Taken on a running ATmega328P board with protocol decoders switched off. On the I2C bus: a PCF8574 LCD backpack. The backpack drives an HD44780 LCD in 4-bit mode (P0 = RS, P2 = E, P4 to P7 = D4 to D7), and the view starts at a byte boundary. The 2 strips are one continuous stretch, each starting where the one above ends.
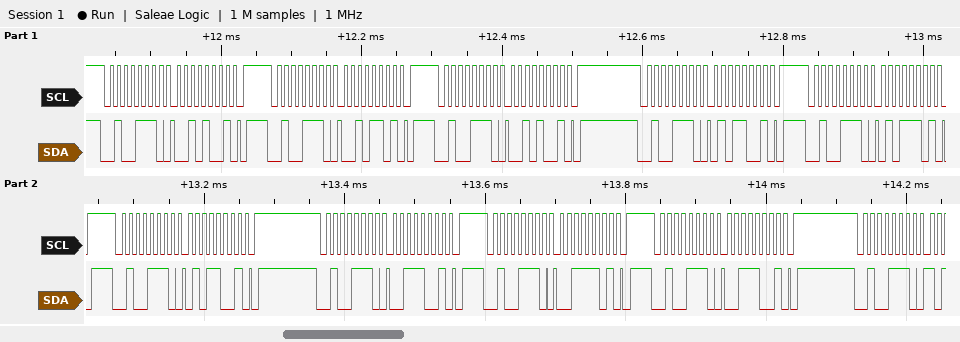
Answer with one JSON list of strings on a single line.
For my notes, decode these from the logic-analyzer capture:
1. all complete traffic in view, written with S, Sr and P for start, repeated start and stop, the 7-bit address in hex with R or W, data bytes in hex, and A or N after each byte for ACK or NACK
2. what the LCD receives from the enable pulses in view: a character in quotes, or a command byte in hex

["S 27W A 29 A P S 27W A 2D A P S 27W A 29 A P S 27W A 59 A P S 27W A 5D A P S 27W A 59 A P S 27W A 39 A P S 27W A 3D A P S 27W A 39 A P S 27W A", "'%'"]
